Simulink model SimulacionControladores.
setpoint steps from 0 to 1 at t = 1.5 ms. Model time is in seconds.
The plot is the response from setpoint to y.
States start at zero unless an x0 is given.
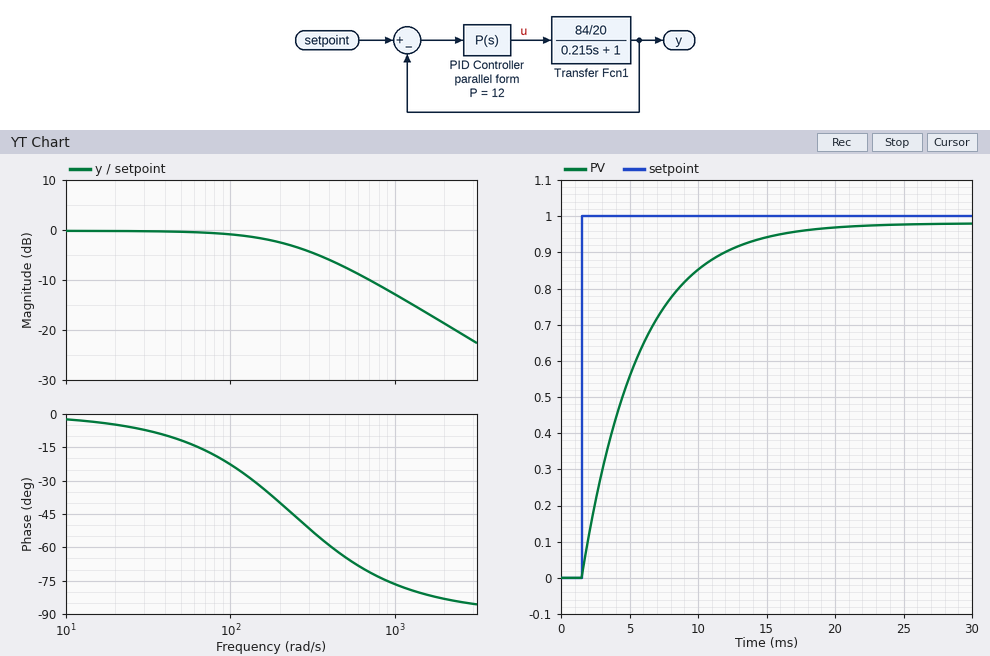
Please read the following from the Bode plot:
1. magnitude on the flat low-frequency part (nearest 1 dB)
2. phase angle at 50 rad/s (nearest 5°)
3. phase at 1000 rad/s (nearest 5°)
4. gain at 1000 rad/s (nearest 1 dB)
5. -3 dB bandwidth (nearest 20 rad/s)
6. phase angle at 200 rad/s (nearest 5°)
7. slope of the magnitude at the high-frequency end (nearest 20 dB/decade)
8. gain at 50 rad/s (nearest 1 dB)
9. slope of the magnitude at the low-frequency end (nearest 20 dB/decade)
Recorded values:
0 dB
-10°
-75°
-13 dB
240 rad/s
-40°
-20 dB/decade
0 dB
0 dB/decade
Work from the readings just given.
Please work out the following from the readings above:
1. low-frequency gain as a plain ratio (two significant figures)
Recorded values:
1.0
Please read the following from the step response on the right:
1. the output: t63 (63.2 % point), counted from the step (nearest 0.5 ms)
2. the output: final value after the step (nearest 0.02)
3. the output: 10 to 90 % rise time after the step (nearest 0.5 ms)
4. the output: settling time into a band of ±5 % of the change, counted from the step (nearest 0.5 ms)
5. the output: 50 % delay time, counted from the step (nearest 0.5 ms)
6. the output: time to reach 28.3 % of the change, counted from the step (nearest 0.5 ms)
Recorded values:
4.0 ms
0.98
9.0 ms
12.5 ms
3.0 ms
1.5 ms
